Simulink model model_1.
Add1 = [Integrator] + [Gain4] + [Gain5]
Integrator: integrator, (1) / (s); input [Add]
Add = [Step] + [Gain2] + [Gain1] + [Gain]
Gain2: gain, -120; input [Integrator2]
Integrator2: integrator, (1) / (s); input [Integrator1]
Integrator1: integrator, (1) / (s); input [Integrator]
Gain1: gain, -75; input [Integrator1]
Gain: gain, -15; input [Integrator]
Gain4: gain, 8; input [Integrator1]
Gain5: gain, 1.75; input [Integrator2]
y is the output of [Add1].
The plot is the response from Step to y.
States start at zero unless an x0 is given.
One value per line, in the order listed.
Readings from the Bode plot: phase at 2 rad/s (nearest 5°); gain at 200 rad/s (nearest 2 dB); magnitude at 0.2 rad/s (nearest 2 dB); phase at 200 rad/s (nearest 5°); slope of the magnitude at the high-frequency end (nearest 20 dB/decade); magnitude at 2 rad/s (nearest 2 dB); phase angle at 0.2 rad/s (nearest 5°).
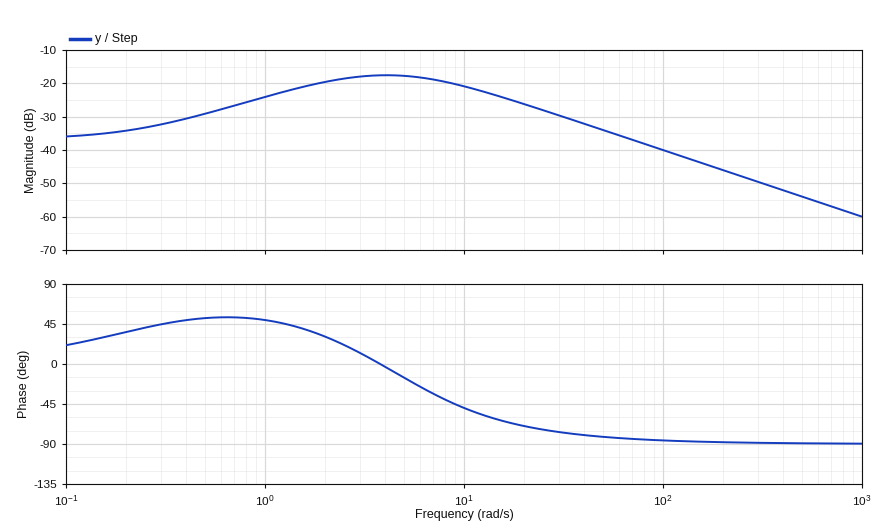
30°
-46 dB
-34 dB
-90°
-20 dB/decade
-20 dB
35°
